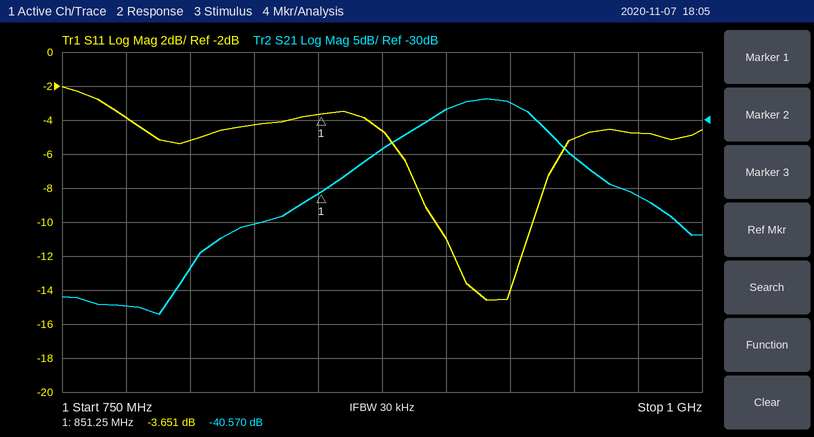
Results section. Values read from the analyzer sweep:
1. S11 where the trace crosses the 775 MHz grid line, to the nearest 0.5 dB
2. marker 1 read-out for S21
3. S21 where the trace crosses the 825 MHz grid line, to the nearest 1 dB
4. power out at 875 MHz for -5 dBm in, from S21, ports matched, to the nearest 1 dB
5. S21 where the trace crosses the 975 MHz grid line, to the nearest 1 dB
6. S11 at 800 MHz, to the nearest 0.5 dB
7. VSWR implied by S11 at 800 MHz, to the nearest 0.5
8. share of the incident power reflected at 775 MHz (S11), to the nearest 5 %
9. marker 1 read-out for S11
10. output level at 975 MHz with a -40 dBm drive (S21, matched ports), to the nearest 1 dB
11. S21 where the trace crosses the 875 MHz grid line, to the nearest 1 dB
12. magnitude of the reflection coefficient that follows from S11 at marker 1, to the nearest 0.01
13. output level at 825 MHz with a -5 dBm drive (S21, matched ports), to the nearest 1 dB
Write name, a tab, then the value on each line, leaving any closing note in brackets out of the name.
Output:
S11 where the trace crosses the 775 MHz grid line, to the nearest 0.5 dB	-4.0 dB
marker 1 read-out for S21	-40.570 dB
S21 where the trace crosses the 825 MHz grid line, to the nearest 1 dB	-45 dB
power out at 875 MHz for -5 dBm in, from S21, ports matched, to the nearest 1 dB	-39 dBm
S21 where the trace crosses the 975 MHz grid line, to the nearest 1 dB	-41 dB
S11 at 800 MHz, to the nearest 0.5 dB	-5.0 dB
VSWR implied by S11 at 800 MHz, to the nearest 0.5	3.5
share of the incident power reflected at 775 MHz (S11), to the nearest 5 %	40 %
marker 1 read-out for S11	-3.651 dB
output level at 975 MHz with a -40 dBm drive (S21, matched ports), to the nearest 1 dB	-81 dBm
S21 where the trace crosses the 875 MHz grid line, to the nearest 1 dB	-34 dB
magnitude of the reflection coefficient that follows from S11 at marker 1, to the nearest 0.01	0.66
output level at 825 MHz with a -5 dBm drive (S21, matched ports), to the nearest 1 dB	-50 dBm
